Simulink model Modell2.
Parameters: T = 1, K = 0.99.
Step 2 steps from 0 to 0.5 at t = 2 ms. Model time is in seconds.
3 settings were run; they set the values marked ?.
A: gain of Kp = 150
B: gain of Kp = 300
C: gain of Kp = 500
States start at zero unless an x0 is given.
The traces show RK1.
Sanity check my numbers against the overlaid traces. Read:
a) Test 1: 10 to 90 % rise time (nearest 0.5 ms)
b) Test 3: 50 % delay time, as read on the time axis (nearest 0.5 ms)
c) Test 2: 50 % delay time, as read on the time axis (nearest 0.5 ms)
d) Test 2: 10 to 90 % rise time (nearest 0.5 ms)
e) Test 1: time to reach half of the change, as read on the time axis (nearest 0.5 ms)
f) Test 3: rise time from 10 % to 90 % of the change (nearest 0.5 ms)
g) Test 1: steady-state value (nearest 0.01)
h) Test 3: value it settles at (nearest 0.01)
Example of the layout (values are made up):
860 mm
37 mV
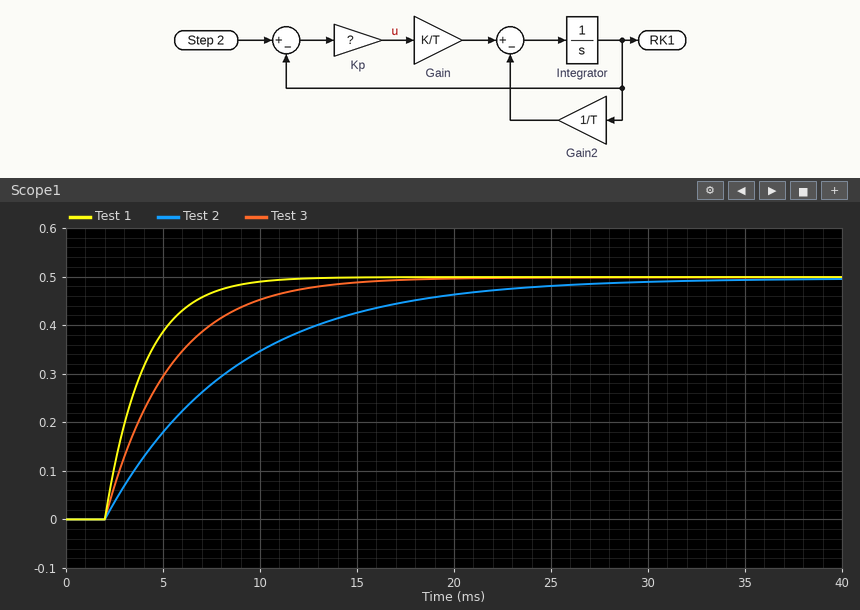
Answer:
4.5 ms
4.5 ms
6.5 ms
14.5 ms
3.5 ms
7.5 ms
0.50
0.50
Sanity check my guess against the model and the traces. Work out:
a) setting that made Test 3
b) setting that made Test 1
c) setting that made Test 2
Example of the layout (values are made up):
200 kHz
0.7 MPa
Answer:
B
C
A
